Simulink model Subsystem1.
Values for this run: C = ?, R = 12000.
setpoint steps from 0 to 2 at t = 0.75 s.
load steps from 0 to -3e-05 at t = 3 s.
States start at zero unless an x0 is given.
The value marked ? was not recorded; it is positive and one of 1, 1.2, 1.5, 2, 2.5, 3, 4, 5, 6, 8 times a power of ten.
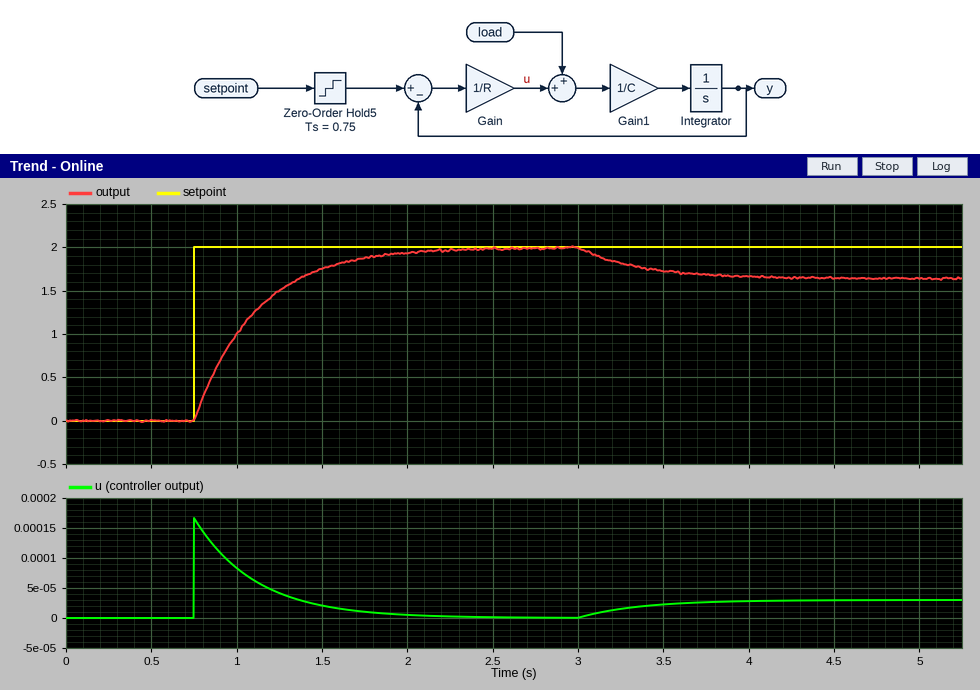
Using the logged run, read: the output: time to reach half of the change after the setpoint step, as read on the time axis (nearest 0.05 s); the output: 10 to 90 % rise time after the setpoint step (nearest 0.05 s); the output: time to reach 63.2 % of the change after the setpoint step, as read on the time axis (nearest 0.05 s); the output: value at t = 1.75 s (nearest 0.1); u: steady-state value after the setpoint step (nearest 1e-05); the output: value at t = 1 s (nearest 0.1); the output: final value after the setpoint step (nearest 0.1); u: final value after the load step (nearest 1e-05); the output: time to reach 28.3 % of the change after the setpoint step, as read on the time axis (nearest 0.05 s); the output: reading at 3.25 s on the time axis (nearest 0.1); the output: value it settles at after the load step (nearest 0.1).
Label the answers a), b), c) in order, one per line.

a) 1.00 s
b) 0.80 s
c) 1.10 s
d) 1.9
e) 0.00000
f) 1.0
g) 2.0
h) 0.00003
i) 0.85 s
j) 1.8
k) 1.6
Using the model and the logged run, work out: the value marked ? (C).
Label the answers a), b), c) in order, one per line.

a) 3e-05
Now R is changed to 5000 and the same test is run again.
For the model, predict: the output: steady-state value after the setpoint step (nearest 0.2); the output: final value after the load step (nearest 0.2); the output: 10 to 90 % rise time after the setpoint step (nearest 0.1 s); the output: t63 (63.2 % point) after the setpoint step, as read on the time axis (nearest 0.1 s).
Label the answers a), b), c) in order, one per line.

a) 2.0
b) 1.8
c) 0.3 s
d) 0.9 s
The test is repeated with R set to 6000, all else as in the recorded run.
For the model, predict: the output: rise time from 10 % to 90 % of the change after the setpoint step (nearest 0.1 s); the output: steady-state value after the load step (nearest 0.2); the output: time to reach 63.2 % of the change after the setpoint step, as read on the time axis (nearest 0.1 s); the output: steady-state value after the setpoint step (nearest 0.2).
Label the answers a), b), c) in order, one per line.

a) 0.4 s
b) 1.8
c) 0.9 s
d) 2.0
